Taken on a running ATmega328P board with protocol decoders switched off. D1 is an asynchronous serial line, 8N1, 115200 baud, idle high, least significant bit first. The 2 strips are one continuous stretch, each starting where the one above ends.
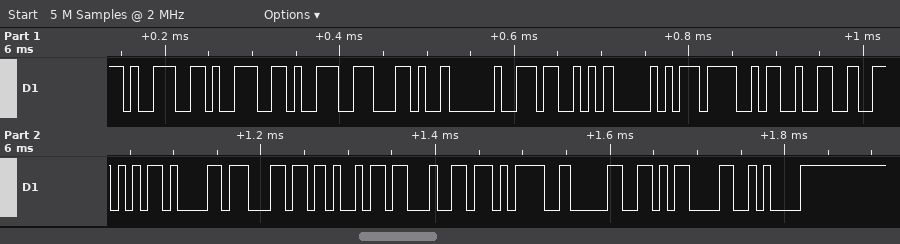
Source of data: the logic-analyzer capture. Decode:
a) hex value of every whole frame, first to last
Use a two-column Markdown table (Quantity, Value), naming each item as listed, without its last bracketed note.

| Quantity | Value |
|---|---|
| hex value of every whole frame, first to last | 0x39 0x39 0x39 0x2C 0x20 0x53 0x50 0x4F 0x32 0x56 0x61 0x6C 0x69 0x64 0x3D 0x30 0x0D 0x0A |
